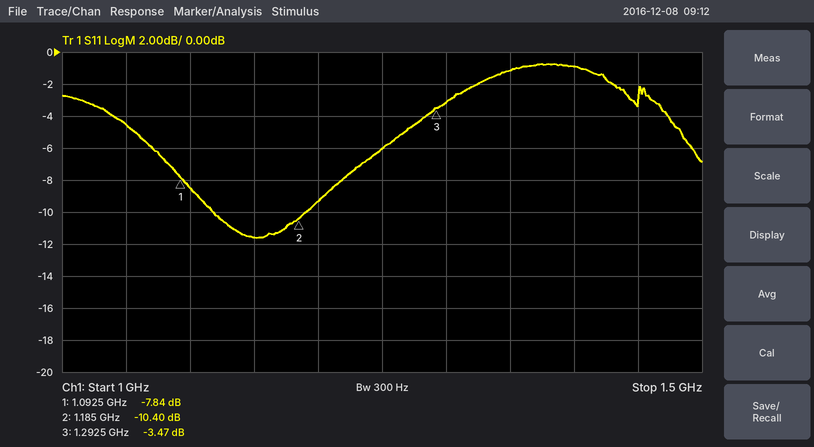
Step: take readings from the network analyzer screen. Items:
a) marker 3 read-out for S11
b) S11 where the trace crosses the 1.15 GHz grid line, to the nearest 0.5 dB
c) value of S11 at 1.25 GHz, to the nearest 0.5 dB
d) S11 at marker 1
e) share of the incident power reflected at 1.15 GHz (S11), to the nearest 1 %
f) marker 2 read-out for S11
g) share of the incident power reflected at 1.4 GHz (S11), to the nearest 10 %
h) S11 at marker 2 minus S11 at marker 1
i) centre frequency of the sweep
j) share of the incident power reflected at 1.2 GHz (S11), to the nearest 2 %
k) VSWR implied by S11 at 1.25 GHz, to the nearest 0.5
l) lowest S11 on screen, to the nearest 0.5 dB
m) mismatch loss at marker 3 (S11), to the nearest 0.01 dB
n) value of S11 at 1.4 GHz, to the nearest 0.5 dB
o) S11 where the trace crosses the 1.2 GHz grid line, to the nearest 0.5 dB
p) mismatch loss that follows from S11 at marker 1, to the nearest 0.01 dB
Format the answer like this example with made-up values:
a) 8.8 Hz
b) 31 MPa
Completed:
a) -3.47 dB
b) -11.5 dB
c) -6.0 dB
d) -7.84 dB
e) 7 %
f) -10.40 dB
g) 80 %
h) -2.56 dB
i) 1.25 GHz
j) 12 %
k) 3.0
l) -11.5 dB
m) 2.59 dB
n) -1.0 dB
o) -9.5 dB
p) 0.78 dB
